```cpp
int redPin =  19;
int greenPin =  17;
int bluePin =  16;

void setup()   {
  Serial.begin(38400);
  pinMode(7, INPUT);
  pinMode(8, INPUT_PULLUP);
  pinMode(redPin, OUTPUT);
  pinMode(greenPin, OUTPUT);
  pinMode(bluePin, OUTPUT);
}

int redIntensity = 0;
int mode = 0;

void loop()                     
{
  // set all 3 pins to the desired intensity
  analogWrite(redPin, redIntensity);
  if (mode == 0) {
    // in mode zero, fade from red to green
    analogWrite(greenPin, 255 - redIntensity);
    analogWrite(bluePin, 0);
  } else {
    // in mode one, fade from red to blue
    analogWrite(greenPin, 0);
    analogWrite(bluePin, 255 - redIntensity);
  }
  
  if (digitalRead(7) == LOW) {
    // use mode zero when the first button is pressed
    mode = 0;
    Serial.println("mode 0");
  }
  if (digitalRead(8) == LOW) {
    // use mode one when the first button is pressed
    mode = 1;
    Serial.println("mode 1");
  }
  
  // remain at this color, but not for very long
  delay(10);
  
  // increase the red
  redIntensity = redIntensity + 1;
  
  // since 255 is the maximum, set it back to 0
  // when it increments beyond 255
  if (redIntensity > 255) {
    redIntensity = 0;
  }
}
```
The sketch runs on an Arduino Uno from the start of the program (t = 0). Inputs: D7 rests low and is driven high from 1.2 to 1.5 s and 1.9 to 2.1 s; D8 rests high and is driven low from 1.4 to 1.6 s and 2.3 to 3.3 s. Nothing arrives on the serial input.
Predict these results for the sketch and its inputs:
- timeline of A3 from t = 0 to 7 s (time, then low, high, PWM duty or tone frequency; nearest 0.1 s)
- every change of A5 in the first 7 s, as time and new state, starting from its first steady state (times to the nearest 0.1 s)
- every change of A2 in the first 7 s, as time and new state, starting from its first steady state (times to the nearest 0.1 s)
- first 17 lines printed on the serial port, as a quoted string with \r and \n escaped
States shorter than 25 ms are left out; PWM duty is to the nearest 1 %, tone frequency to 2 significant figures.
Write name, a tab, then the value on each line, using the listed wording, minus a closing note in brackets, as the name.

timeline of A3 from t = 0 to 7 s	0 s high; 1.3 s low; 3.3 s high; 3.9 s low; 5.2 s high; 6.5 s low
every change of A5 in the first 7 s, as time and new state, starting from its first steady state	0 s low; 1.3 s high; 2.6 s low; 3.9 s high; 5.2 s low; 6.5 s high
every change of A2 in the first 7 s, as time and new state, starting from its first steady state	0 s low; 2.6 s high; 3.3 s low
first 17 lines printed on the serial port, as a quoted string with \r and \n escaped	"mode 0\r\nmode 0\r\nmode 0\r\nmode 0\r\nmode 0\r\nmode 0\r\nmode 0\r\nmode 0\r\nmode 0\r\nmode 0\r\nmode 0\r\nmode 0\r\nmode 0\r\nmode 0\r\nmode 0\r\nmode 0\r\nmode 0\r\n"
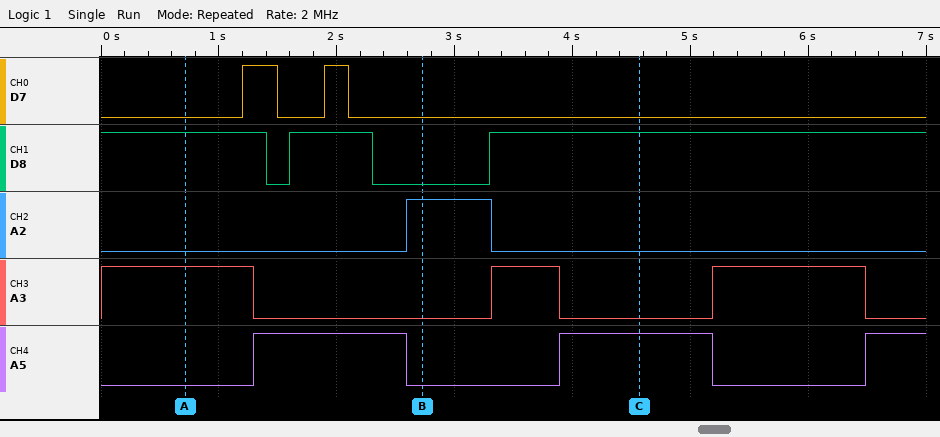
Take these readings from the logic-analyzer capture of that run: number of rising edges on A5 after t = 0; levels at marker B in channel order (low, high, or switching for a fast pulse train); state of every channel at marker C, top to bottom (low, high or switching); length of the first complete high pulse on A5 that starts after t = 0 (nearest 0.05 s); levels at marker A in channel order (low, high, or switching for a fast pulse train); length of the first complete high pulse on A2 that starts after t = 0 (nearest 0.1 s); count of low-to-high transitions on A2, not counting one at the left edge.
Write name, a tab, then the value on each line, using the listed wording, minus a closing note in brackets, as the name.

number of rising edges on A5 after t = 0	3
levels at marker B in channel order	D7 low, D8 low, A2 high, A3 low, A5 low
state of every channel at marker C, top to bottom	D7 low, D8 high, A2 low, A3 low, A5 high
length of the first complete high pulse on A5 that starts after t = 0	1.30 s
levels at marker A in channel order	D7 low, D8 high, A2 low, A3 high, A5 low
length of the first complete high pulse on A2 that starts after t = 0	0.7 s
count of low-to-high transitions on A2, not counting one at the left edge	1
